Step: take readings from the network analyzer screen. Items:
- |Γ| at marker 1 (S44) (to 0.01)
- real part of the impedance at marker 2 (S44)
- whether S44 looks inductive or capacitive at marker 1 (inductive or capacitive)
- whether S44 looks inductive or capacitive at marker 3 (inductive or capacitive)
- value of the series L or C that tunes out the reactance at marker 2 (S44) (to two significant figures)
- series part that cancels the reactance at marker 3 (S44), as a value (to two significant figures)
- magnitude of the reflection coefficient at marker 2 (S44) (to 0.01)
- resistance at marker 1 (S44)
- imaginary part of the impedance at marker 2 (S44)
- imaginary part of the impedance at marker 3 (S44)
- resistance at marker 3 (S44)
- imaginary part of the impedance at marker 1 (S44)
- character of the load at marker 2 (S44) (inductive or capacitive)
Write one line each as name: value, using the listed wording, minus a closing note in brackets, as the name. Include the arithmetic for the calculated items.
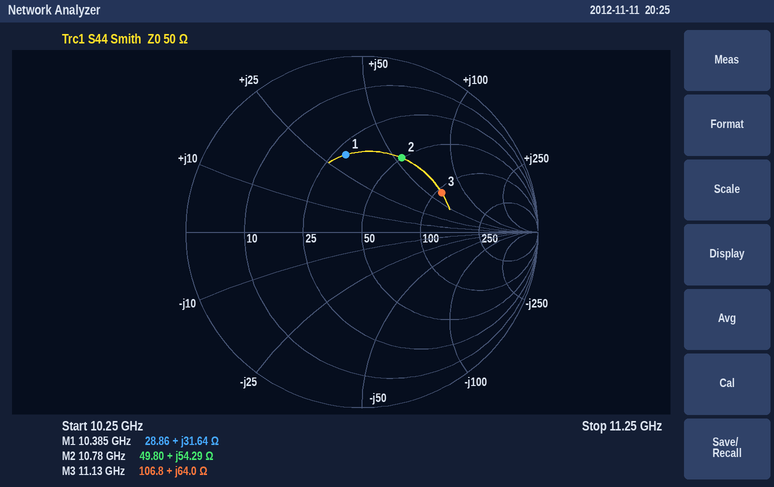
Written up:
|Γ| at marker 1 (S44): 0.45
real part of the impedance at marker 2: 49.80 Ω
whether S44 looks inductive or capacitive at marker 1: inductive
whether S44 looks inductive or capacitive at marker 3: inductive
value of the series L or C that tunes out the reactance at marker 2 (S44): C = 1/(2π × 10.78 GHz × 54.29 Ω) ≈ 272 fF, so 270 fF to two significant figures
series part that cancels the reactance at marker 3 (S44), as a value: C = 1/(2π × 11.13 GHz × 64 Ω) ≈ 223 fF, so 220 fF to two significant figures
magnitude of the reflection coefficient at marker 2 (S44): 0.48
resistance at marker 1: 28.86 Ω
imaginary part of the impedance at marker 2: +54.29 Ω
imaginary part of the impedance at marker 3: +64.0 Ω
resistance at marker 3: 106.8 Ω
imaginary part of the impedance at marker 1: +31.64 Ω
character of the load at marker 2 (S44): inductive
